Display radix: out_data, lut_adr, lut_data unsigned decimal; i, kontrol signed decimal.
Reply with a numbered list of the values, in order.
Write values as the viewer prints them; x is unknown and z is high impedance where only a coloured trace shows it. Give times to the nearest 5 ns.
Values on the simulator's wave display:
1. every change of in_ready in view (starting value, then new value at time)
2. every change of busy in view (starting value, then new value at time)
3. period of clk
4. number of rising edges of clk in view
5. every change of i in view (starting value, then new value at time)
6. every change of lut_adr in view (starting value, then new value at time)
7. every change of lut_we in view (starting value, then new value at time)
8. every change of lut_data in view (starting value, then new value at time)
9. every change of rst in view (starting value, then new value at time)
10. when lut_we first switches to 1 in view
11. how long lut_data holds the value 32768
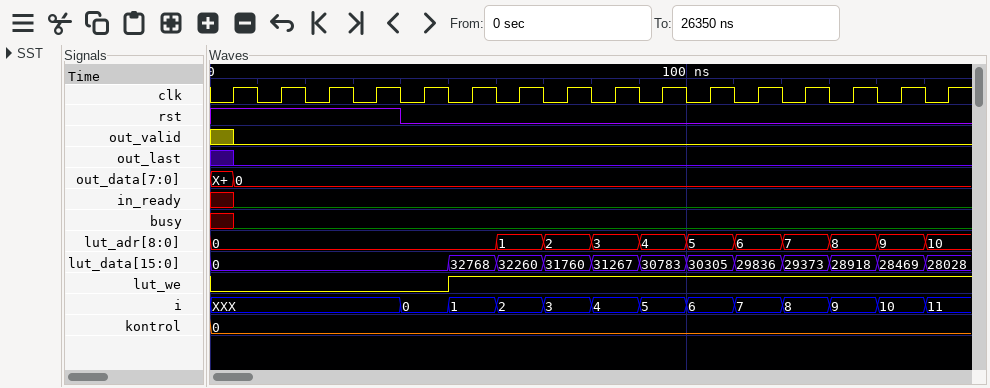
1. x, 0 at 5 ns
2. x, 0 at 5 ns
3. 10 ns
4. 16
5. XXX, 0 at 40 ns, 1 at 50 ns, 2 at 60 ns, 3 at 70 ns, 4 at 80 ns, 5 at 90 ns, 6 at 100 ns, 7 at 110 ns, 8 at 120 ns, 9 at 130 ns, 10 at 140 ns, 11 at 150 ns
6. 0, 1 at 60 ns, 2 at 70 ns, 3 at 80 ns, 4 at 90 ns, 5 at 100 ns, 6 at 110 ns, 7 at 120 ns, 8 at 130 ns, 9 at 140 ns, 10 at 150 ns
7. 0, 1 at 50 ns
8. 0, 32768 at 50 ns, 32260 at 60 ns, 31760 at 70 ns, 31267 at 80 ns, 30783 at 90 ns, 30305 at 100 ns, 29836 at 110 ns, 29373 at 120 ns, 28918 at 130 ns, 28469 at 140 ns, 28028 at 150 ns
9. 1, 0 at 40 ns
10. 50 ns
11. 10 ns
